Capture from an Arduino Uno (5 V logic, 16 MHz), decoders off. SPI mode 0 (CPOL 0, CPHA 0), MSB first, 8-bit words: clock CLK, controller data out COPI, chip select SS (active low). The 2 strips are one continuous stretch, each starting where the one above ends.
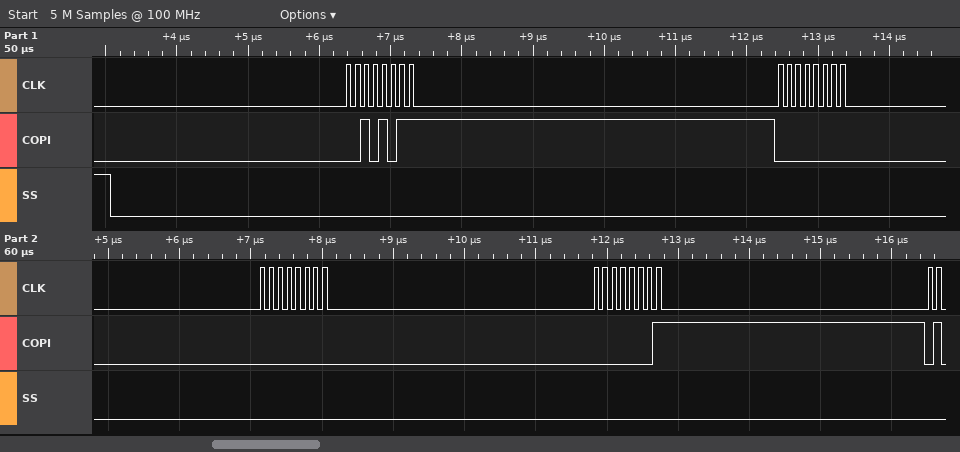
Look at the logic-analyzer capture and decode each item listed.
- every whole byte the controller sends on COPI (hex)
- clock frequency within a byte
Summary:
2B 00 00 01
8 MHz
